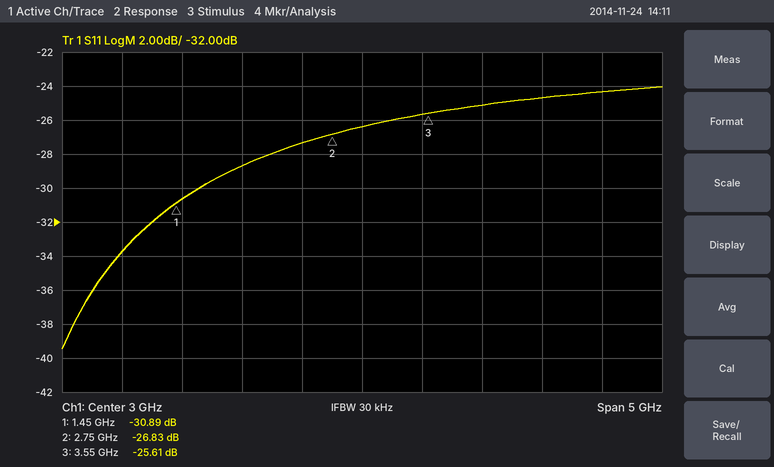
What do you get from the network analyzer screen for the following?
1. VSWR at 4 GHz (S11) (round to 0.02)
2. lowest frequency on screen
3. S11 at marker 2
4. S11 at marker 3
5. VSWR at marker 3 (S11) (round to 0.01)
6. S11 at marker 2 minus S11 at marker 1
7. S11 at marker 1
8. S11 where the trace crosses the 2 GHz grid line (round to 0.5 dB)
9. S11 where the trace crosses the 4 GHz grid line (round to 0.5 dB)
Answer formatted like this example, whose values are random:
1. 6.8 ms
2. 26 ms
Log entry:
1. 1.12
2. 500 MHz
3. -26.83 dB
4. -25.61 dB
5. 1.11
6. 4.06 dB
7. -30.89 dB
8. -28.5 dB
9. -25.0 dB
